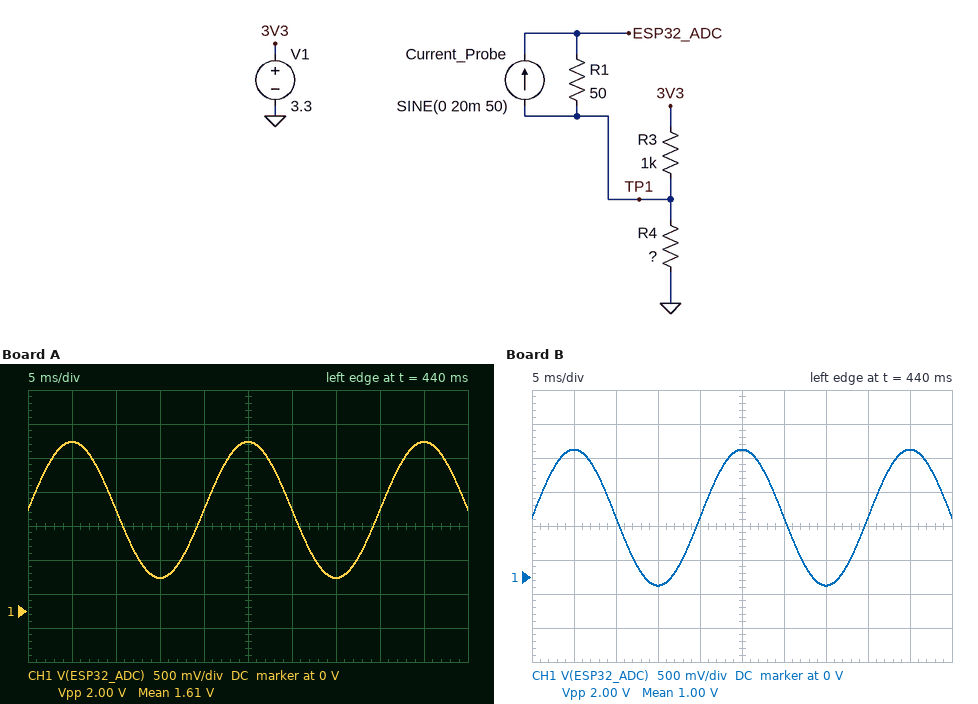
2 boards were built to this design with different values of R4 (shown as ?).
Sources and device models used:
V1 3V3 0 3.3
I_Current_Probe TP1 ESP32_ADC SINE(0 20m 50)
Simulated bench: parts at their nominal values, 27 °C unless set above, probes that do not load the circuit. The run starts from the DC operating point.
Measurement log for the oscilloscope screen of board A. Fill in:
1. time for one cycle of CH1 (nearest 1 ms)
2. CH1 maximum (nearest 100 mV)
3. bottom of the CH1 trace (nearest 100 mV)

20 ms
2.5 V
500 mV
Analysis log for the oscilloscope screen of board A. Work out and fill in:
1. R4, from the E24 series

820 Ω
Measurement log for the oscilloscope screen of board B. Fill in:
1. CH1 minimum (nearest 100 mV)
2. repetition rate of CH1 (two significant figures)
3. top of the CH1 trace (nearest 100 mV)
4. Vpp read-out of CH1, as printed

-100 mV
50 Hz
1.9 V
2.00 V
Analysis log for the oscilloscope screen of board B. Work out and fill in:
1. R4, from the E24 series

360 Ω
